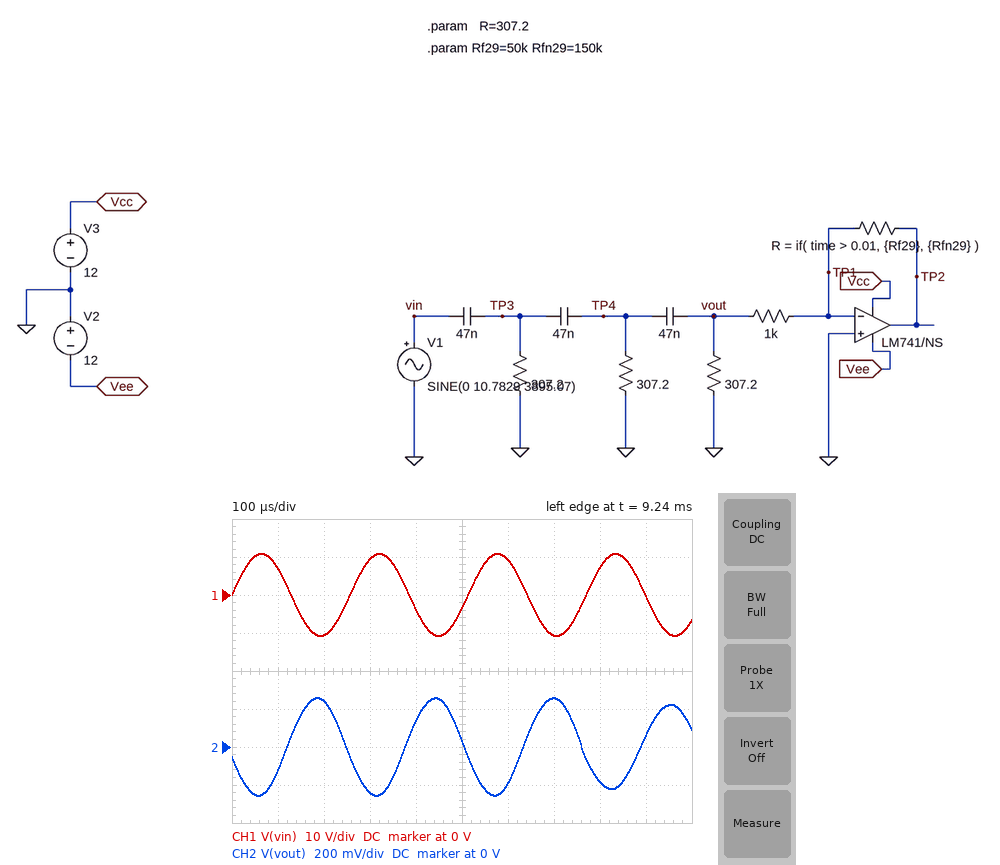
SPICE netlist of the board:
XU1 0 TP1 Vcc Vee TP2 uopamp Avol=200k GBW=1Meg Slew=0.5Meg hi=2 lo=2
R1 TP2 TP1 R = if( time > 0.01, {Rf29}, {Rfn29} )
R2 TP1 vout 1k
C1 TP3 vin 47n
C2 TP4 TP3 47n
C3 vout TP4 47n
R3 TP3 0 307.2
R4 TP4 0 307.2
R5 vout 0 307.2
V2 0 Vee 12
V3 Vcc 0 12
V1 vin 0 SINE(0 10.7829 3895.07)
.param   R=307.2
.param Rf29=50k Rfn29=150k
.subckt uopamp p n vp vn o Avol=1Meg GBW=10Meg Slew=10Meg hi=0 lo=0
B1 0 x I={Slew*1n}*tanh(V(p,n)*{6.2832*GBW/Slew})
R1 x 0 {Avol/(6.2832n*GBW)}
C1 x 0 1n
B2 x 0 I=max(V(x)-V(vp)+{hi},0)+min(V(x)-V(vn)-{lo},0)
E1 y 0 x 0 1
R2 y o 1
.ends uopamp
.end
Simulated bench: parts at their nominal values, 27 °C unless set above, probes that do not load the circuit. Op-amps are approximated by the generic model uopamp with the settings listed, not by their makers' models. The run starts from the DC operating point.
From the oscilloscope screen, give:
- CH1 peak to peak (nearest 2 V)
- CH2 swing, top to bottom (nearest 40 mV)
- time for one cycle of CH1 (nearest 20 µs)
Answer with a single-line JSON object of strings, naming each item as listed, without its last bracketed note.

{"CH1 peak to peak": "22 V", "CH2 swing, top to bottom": "520 mV", "time for one cycle of CH1": "260 µs"}
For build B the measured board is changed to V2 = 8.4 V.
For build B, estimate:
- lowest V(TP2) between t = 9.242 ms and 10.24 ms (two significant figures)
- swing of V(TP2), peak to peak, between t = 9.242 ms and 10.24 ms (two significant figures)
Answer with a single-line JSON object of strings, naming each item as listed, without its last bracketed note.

{"lowest V(TP2) between t = 9.242 ms and 10.24 ms": "-6.4 V", "swing of V(TP2), peak to peak, between t = 9.242 ms and 10.24 ms": "16 V"}
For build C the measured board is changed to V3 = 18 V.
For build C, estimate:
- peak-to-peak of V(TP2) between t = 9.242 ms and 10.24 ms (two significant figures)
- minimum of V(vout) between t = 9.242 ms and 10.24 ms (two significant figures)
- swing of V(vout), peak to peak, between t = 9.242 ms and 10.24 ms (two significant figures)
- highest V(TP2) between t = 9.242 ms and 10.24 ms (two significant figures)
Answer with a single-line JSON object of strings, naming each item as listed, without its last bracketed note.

{"peak-to-peak of V(TP2) between t = 9.242 ms and 10.24 ms": "26 V", "minimum of V(vout) between t = 9.242 ms and 10.24 ms": "-250 mV", "swing of V(vout), peak to peak, between t = 9.242 ms and 10.24 ms": "500 mV", "highest V(TP2) between t = 9.242 ms and 10.24 ms": "16 V"}
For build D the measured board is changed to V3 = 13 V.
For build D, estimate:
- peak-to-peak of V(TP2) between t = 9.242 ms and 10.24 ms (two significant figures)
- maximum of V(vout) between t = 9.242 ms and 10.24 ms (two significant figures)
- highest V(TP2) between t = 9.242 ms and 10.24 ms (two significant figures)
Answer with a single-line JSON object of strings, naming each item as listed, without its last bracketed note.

{"peak-to-peak of V(TP2) between t = 9.242 ms and 10.24 ms": "21 V", "maximum of V(vout) between t = 9.242 ms and 10.24 ms": "260 mV", "highest V(TP2) between t = 9.242 ms and 10.24 ms": "11 V"}
